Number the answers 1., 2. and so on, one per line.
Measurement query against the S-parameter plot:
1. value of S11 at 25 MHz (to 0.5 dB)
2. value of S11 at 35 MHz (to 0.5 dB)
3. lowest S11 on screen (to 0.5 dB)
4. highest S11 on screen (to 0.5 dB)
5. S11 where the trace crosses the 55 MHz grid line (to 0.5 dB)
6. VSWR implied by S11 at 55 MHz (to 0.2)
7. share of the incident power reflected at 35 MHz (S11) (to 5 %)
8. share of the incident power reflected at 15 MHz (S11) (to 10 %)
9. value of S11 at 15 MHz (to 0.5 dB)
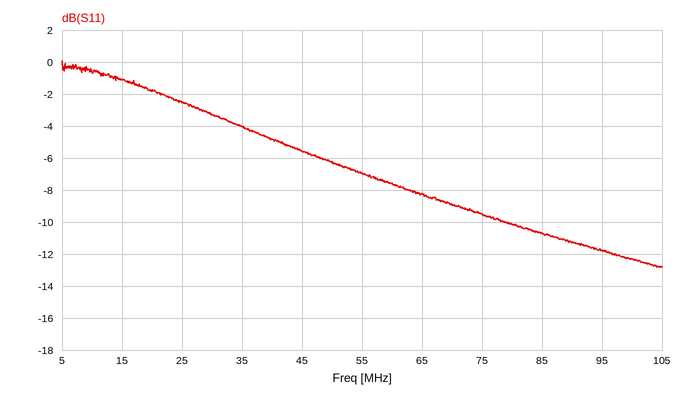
1. -2.5 dB
2. -4.0 dB
3. -13.0 dB
4. 0.0 dB
5. -7.0 dB
6. 2.6
7. 40 %
8. 80 %
9. -1.0 dB
